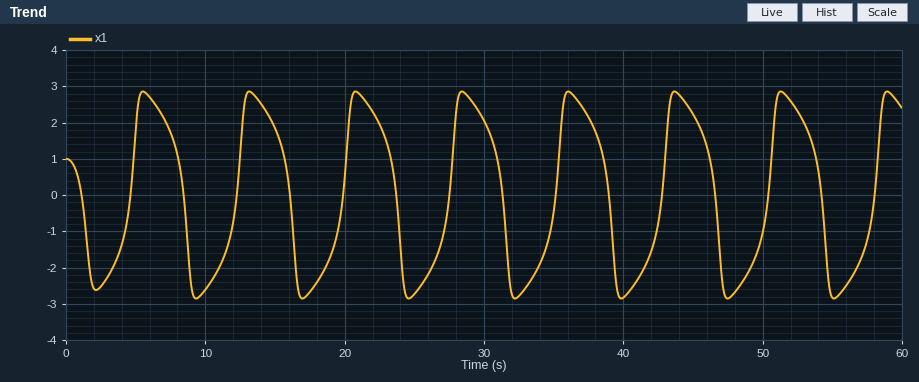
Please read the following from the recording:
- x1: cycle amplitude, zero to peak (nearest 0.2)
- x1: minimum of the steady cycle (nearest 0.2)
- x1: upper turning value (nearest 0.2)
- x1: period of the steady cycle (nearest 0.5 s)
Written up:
2.8
-2.8
2.8
7.5 s
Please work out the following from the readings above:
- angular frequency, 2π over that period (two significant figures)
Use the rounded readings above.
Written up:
0.84 rad/s
